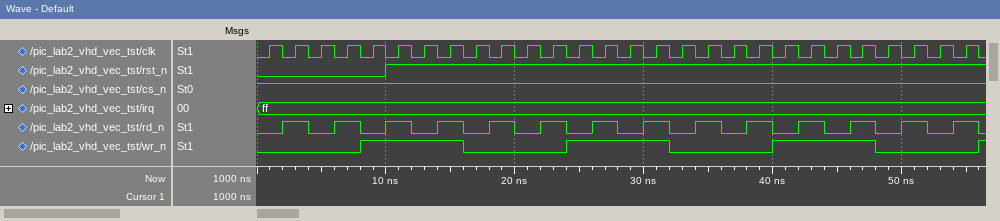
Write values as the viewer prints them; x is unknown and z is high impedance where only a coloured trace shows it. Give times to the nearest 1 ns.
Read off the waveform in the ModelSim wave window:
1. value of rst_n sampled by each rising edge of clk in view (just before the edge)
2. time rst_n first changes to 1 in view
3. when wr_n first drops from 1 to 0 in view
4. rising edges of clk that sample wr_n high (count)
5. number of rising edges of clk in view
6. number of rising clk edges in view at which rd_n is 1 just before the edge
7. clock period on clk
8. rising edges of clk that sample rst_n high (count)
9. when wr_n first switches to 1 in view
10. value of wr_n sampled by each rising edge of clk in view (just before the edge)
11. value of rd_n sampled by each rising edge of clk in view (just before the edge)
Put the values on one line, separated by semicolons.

0 0 0 0 0 1 1 1 1 1 1 1 1 1 1 1 1 1 1 1 1 1 1 1 1 1 1 1; 10 ns; 16 ns; 12; 28; 14; 2 ns; 23; 8 ns; 0 0 0 0 1 1 1 1 0 0 0 0 1 1 1 1 0 0 0 0 1 1 1 1 0 0 0 0; 0 1 0 1 0 1 0 1 0 1 0 1 0 1 0 1 0 1 0 1 0 1 0 1 0 1 0 1
